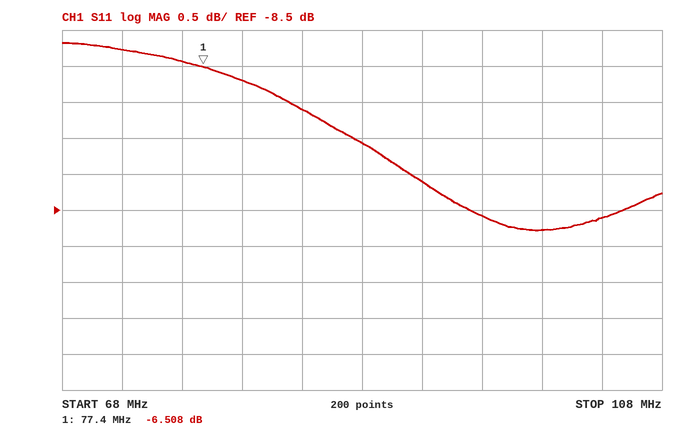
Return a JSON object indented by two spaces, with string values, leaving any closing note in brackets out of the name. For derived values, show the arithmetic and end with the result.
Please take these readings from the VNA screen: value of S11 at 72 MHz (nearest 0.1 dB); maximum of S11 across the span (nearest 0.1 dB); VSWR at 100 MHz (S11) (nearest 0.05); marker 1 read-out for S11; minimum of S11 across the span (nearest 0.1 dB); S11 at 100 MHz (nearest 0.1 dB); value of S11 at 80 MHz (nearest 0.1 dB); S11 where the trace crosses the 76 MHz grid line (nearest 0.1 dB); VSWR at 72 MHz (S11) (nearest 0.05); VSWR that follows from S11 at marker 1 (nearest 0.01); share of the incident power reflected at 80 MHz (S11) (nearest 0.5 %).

{
  "value of S11 at 72 MHz": "-6.3 dB",
  "maximum of S11 across the span": "-6.2 dB",
  "VSWR at 100 MHz (S11)": "|Γ| = 10^(-8.8/20) = 0.3631; VSWR = (1 + 0.3631)/(1 − 0.3631) ≈ 2.14, so 2.15 to the nearest 0.05",
  "marker 1 read-out for S11": "-6.508 dB",
  "minimum of S11 across the span": "-8.8 dB",
  "S11 at 100 MHz": "-8.8 dB",
  "value of S11 at 80 MHz": "-6.7 dB",
  "S11 where the trace crosses the 76 MHz grid line": "-6.4 dB",
  "VSWR at 72 MHz (S11)": "|Γ| = 10^(-6.3/20) = 0.4842; VSWR = (1 + 0.4842)/(1 − 0.4842) ≈ 2.88, so 2.90 to the nearest 0.05",
  "VSWR that follows from S11 at marker 1": "(1 + 0.4727)/(1 − 0.4727) ≈ 2.79",
  "share of the incident power reflected at 80 MHz (S11)": "10^(-6.7/10) ≈ 21.4 %, so 21.5 % to the nearest 0.5 %"
}
